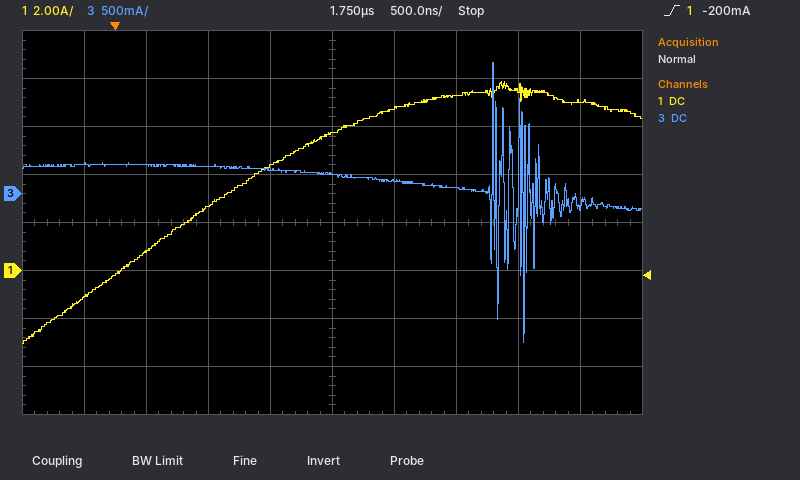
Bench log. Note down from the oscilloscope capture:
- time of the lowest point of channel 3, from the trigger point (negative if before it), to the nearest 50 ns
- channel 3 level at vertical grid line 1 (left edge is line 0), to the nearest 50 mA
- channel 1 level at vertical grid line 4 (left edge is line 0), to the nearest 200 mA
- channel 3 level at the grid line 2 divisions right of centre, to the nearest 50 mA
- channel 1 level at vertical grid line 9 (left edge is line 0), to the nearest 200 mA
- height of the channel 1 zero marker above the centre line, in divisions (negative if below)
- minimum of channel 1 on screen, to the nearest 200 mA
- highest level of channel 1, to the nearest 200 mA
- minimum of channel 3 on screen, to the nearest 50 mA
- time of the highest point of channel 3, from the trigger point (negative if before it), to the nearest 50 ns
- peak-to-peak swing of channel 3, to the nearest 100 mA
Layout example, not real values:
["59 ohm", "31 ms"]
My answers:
["+3.30 µs", "300 mA", "4.4 A", "50 mA", "7.0 A", "-1.0 div", "-3.0 A", "7.8 A", "-1.55 A", "+3.05 µs", "2.90 A"]
